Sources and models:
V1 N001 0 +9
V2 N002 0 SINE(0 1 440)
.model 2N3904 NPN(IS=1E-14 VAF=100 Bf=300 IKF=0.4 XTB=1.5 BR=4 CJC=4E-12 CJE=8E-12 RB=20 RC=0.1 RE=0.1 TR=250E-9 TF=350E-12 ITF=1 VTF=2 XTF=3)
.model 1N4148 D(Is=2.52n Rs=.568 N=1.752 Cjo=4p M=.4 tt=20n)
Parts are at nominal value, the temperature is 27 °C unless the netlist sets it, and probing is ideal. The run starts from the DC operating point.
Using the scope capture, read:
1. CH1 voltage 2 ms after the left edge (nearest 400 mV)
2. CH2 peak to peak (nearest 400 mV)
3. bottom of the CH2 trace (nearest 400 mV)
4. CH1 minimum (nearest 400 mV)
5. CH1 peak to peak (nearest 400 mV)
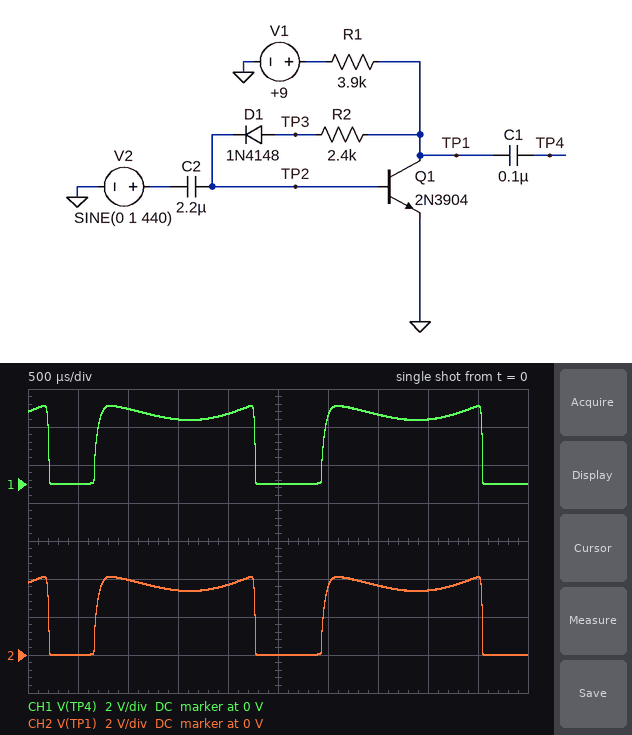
3.6 V
4.0 V
0 V
0 V
4.0 V
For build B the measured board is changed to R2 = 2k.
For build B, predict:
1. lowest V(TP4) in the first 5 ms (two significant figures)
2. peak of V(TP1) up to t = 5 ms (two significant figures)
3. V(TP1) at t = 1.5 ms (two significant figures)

9.4 mV
3.8 V
3.0 V
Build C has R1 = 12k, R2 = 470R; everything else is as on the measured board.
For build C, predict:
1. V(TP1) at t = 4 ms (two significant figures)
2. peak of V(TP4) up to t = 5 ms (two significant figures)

-49 mV
1.4 V
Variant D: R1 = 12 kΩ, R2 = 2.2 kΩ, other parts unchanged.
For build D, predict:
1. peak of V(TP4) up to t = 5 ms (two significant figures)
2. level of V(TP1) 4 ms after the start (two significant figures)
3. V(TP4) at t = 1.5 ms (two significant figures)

2.3 V
1.0 V
1.1 V
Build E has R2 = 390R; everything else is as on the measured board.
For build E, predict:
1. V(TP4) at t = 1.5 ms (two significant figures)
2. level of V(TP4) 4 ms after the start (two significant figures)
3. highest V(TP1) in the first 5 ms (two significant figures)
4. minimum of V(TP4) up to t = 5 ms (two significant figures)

980 mV
1.0 V
1.9 V
9.4 mV
